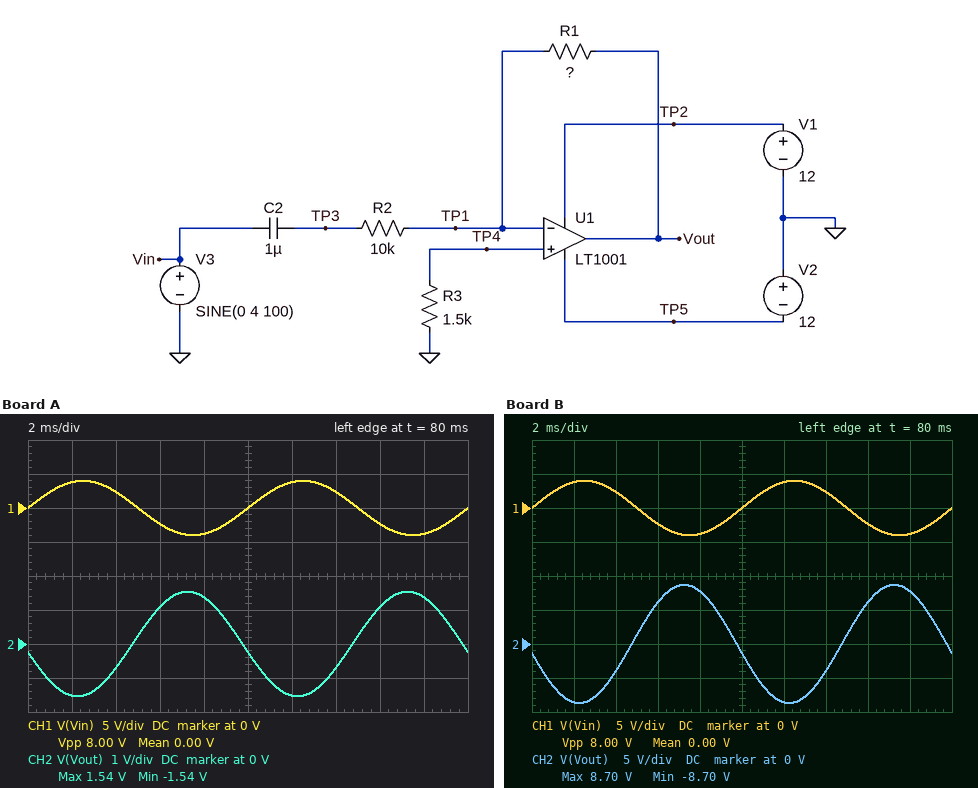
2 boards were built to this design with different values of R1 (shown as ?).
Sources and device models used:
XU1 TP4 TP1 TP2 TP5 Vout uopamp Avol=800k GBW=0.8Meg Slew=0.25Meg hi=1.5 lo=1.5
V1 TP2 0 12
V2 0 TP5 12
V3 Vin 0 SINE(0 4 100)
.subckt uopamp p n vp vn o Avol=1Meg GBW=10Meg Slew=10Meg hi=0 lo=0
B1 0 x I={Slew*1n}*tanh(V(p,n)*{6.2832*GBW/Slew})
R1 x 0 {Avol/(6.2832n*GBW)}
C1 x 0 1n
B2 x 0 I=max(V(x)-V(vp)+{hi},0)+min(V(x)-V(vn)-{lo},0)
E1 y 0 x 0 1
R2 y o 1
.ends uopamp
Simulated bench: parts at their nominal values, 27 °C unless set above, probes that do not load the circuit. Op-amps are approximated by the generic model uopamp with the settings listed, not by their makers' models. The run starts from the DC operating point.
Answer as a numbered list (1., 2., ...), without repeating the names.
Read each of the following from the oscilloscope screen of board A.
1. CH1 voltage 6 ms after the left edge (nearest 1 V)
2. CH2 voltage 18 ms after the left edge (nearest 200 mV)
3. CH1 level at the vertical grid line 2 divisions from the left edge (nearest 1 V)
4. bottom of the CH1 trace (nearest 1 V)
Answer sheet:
1. -2 V
2. 1.4 V
3. 2 V
4. -4 V
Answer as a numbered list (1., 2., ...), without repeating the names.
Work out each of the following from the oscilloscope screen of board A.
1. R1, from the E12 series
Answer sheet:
1. 3.9 kΩ
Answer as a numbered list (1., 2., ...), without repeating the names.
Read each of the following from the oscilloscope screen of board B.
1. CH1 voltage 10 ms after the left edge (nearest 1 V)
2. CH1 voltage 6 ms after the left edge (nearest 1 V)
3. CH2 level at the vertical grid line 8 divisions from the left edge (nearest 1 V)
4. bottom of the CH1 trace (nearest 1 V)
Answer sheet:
1. 0 V
2. -2 V
3. 6 V
4. -4 V
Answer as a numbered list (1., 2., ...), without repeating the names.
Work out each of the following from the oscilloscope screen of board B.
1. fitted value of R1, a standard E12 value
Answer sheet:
1. 22 kΩ
